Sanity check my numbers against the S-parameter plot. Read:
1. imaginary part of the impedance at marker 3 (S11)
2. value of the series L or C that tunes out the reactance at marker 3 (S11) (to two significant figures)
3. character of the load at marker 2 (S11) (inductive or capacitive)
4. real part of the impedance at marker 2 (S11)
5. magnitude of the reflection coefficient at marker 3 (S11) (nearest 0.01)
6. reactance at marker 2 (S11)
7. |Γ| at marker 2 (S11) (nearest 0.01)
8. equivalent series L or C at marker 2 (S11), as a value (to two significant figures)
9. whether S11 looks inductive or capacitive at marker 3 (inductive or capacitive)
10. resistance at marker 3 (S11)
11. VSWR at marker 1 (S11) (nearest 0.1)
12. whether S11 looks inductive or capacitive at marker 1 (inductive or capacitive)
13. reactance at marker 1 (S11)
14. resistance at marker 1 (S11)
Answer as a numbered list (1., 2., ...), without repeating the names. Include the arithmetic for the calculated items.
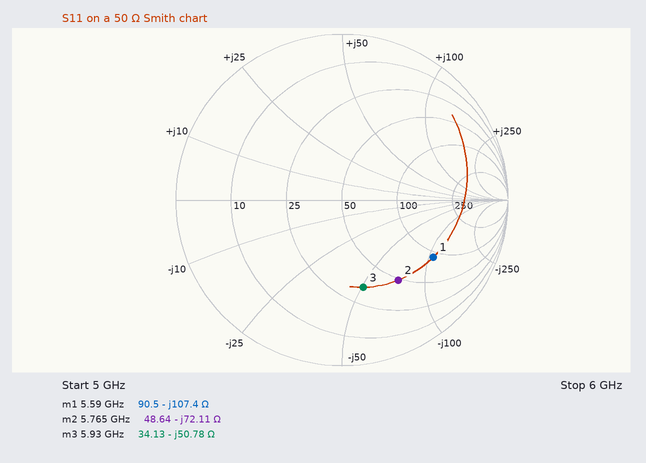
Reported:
1. -50.78 Ω
2. L = 50.78 Ω/(2π × 5.93 GHz) ≈ 1.4 nH
3. capacitive
4. 48.64 Ω
5. 0.54
6. -72.11 Ω
7. 0.59
8. C = 1/(2π × 5.765 GHz × 72.11 Ω) ≈ 383 fF, so 380 fF to two significant figures
9. capacitive
10. 34.13 Ω
11. 4.7
12. capacitive
13. -107.4 Ω
14. 90.5 Ω
